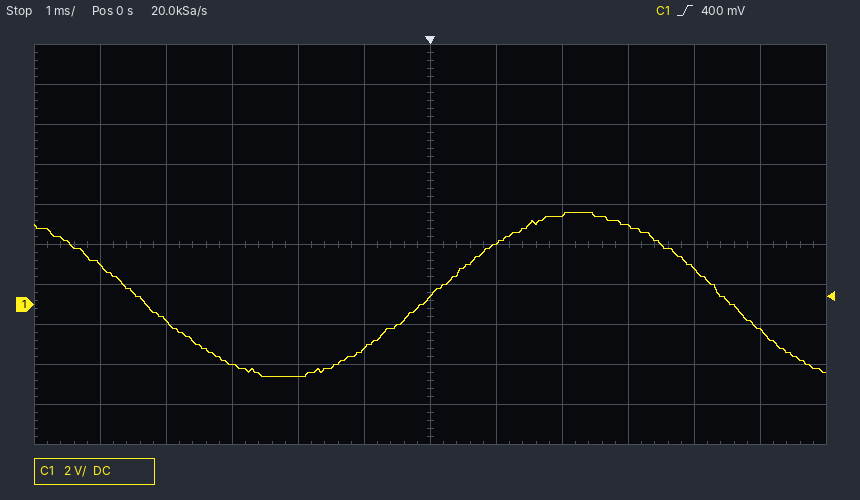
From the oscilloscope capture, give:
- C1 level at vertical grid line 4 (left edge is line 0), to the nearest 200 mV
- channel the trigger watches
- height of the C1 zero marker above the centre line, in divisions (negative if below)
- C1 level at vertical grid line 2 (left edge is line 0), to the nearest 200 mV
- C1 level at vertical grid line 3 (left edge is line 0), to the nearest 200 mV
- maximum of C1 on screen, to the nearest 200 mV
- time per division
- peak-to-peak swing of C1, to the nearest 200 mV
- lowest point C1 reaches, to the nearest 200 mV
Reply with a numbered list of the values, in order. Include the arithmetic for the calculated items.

1. -3.6 V
2. C1
3. -1.5 div
4. -800 mV
5. -3.0 V
6. 4.6 V
7. 1 ms
8. 4.6 V − (-3.6 V) = 8.2 V
9. -3.6 V
